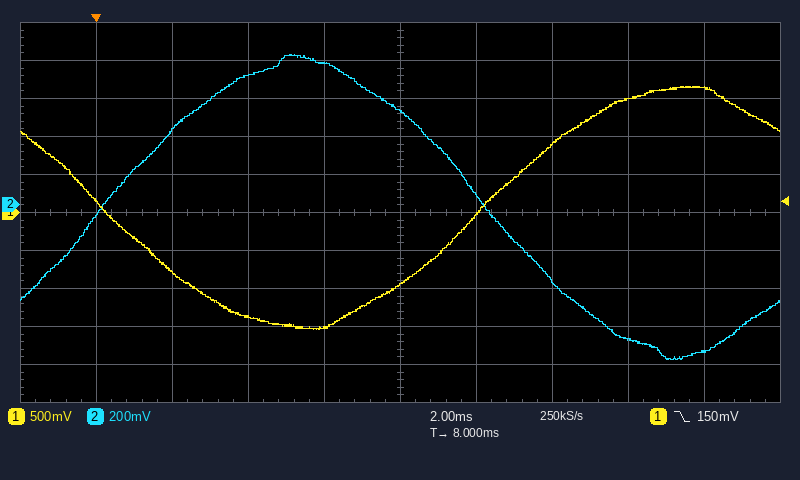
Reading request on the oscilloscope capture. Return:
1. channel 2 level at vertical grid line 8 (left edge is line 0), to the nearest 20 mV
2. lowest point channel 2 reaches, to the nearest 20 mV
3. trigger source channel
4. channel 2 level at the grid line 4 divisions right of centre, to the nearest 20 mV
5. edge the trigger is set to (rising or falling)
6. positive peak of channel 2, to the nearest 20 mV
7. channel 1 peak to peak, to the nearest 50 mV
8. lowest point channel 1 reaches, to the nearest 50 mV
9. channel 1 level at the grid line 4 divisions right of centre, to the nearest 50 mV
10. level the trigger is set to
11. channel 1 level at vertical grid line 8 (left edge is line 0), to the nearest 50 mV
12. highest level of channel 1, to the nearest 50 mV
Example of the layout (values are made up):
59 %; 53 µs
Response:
-700 mV; -820 mV; channel 1; -780 mV; falling; 800 mV; 3.20 V; -1.55 V; 1.65 V; 150 mV; 1.50 V; 1.65 V
